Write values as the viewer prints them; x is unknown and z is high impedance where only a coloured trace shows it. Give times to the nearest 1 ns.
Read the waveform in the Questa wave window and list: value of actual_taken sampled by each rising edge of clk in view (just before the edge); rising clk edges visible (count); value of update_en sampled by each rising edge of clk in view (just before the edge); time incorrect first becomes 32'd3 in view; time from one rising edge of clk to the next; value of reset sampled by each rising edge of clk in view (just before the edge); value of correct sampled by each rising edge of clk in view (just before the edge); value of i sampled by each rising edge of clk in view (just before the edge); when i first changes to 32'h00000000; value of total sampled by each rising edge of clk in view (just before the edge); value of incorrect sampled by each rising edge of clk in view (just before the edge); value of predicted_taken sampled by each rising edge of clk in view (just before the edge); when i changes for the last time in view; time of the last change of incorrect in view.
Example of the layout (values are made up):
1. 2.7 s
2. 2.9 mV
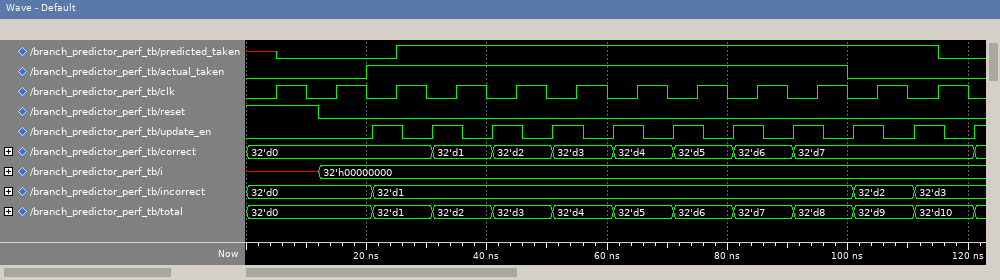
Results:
1. 0 0 1 1 1 1 1 1 1 1 0 0
2. 12
3. 0 0 1 1 1 1 1 1 1 1 1 1
4. 111 ns
5. 10 ns
6. 1 0 0 0 0 0 0 0 0 0 0 0
7. 32'd0, 32'd0, 32'd0, 32'd1, 32'd2, 32'd3, 32'd4, 32'd5, 32'd6, 32'd7, 32'd7, 32'd7
8. x, 32'h00000000, 32'h00000000, 32'h00000000, 32'h00000000, 32'h00000000, 32'h00000000, 32'h00000000, 32'h00000000, 32'h00000000, 32'h00000000, 32'h00000000
9. 12 ns
10. 32'd0, 32'd0, 32'd1, 32'd2, 32'd3, 32'd4, 32'd5, 32'd6, 32'd7, 32'd8, 32'd9, 32'd10
11. 32'd0, 32'd0, 32'd1, 32'd1, 32'd1, 32'd1, 32'd1, 32'd1, 32'd1, 32'd1, 32'd2, 32'd3
12. x 0 0 1 1 1 1 1 1 1 1 1
13. 12 ns
14. 111 ns
